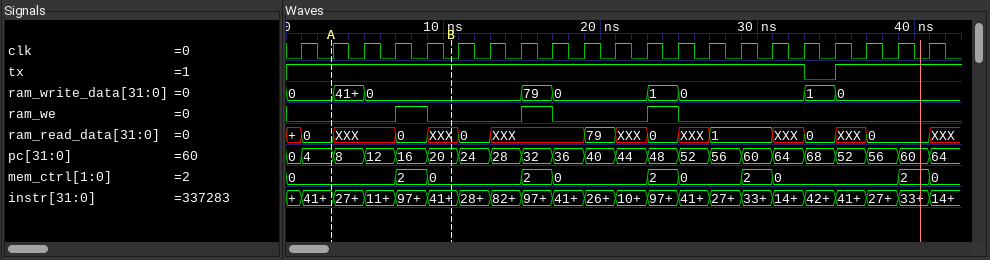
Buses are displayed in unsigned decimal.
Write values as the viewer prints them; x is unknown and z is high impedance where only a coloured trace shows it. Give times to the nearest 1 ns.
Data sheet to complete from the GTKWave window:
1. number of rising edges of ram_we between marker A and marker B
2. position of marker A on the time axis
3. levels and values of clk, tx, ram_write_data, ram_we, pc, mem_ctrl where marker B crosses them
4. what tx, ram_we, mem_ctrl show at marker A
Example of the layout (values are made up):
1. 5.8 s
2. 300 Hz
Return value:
1. 1
2. 3 ns
3. clk=0, tx=1, ram_write_data=0, ram_we=0, pc=20, mem_ctrl=0
4. tx=1, ram_we=0, mem_ctrl=0
